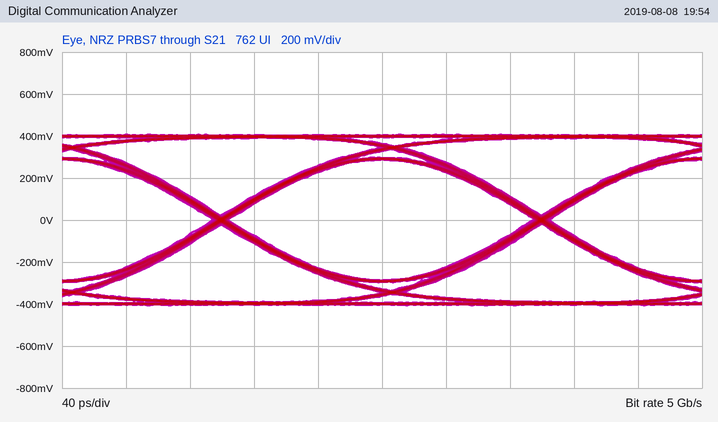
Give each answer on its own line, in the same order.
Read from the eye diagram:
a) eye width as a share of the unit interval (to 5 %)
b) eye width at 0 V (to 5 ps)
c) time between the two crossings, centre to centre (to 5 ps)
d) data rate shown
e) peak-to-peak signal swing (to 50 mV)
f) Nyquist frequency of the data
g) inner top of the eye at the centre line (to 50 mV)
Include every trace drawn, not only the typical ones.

95 %
190 ps
200 ps
5 Gb/s
800 mV
2.5 GHz
300 mV
